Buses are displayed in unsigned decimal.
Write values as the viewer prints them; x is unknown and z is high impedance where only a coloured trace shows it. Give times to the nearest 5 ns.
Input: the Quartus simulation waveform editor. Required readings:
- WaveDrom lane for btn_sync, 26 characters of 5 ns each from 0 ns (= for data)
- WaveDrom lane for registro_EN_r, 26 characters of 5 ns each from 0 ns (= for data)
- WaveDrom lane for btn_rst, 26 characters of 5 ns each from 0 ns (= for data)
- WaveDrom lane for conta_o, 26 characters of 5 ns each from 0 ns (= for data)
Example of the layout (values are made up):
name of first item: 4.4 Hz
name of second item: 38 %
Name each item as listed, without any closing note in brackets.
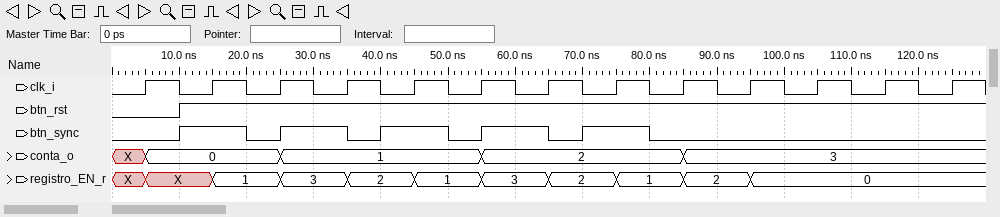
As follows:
WaveDrom lane for btn_sync, 26 characters of 5 ns each from 0 ns: {name: 'btn_sync', wave: '0.1.01.01.01.01.0.........'}
WaveDrom lane for registro_EN_r, 26 characters of 5 ns each from 0 ns: {name: 'registro_EN_r', wave: 'x=.=.=.=.=.=.=.=.=.=......', data: 'X 1 3 2 1 3 2 1 2 0'}
WaveDrom lane for btn_rst, 26 characters of 5 ns each from 0 ns: {name: 'btn_rst', wave: '0.1.......................'}
WaveDrom lane for conta_o, 26 characters of 5 ns each from 0 ns: {name: 'conta_o', wave: 'x=...=.....=.....=........', data: '0 1 2 3'}
